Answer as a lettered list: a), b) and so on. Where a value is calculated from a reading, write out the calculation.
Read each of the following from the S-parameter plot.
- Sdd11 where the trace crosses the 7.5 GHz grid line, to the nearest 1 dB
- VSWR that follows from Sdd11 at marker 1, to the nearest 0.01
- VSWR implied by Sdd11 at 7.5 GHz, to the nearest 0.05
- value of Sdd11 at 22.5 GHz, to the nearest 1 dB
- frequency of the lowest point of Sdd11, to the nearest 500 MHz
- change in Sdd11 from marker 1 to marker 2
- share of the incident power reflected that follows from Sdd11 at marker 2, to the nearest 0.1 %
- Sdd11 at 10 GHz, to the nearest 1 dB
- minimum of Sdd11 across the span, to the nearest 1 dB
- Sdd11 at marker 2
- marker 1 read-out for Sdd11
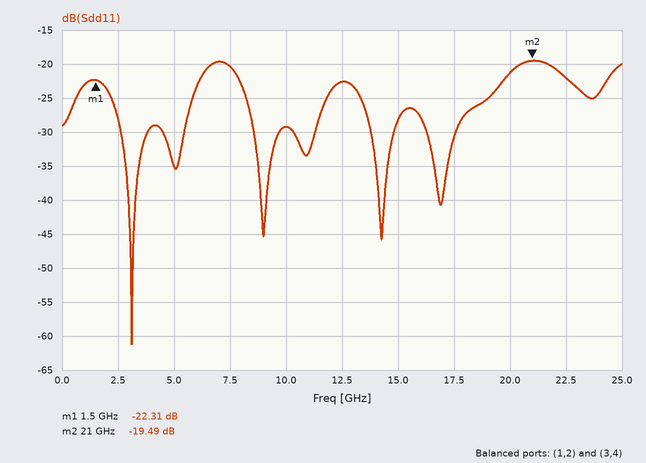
a) -20 dB
b) (1 + 0.0766)/(1 − 0.0766) ≈ 1.17
c) |Γ| = 10^(-20/20) = 0.1000; VSWR = (1 + 0.1000)/(1 − 0.1000) ≈ 1.22, so 1.20 to the nearest 0.05
d) -22 dB
e) 3.0 GHz
f) -19.49 − (-22.31) = 2.82 dB
g) 10^(-19.49/10) ≈ 1.1 %
h) -29 dB
i) -61 dB
j) -19.49 dB
k) -22.31 dB
